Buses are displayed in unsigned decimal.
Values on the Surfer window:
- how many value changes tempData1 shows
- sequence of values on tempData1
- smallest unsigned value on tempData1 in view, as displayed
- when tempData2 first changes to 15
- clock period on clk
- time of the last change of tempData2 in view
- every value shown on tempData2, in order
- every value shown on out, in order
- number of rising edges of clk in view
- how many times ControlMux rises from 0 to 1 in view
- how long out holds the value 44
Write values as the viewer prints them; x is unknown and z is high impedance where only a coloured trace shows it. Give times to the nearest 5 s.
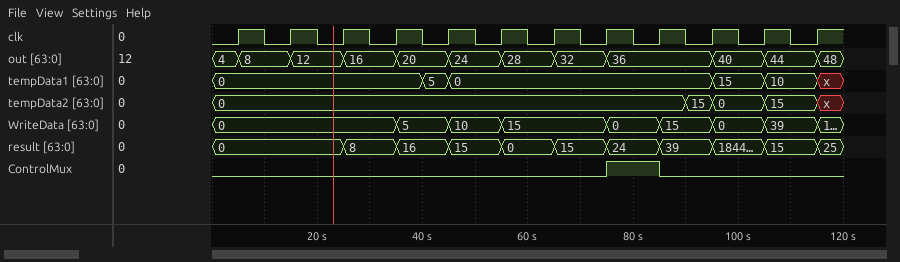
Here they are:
5
0, 5, 0, 15, 10, x
0
90 s
10 s
115 s
0, 15, 0, 15, x
4, 8, 12, 16, 20, 24, 28, 32, 36, 40, 44, 48
12
1
10 s
